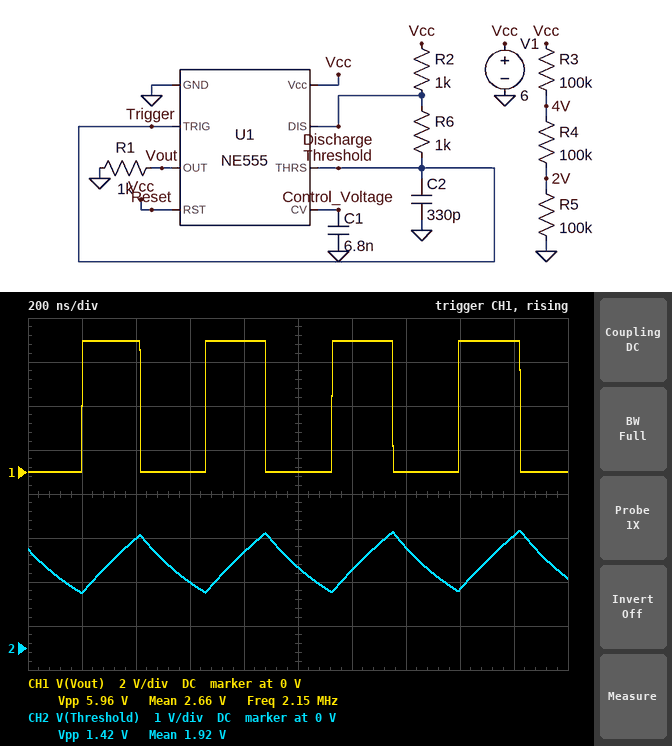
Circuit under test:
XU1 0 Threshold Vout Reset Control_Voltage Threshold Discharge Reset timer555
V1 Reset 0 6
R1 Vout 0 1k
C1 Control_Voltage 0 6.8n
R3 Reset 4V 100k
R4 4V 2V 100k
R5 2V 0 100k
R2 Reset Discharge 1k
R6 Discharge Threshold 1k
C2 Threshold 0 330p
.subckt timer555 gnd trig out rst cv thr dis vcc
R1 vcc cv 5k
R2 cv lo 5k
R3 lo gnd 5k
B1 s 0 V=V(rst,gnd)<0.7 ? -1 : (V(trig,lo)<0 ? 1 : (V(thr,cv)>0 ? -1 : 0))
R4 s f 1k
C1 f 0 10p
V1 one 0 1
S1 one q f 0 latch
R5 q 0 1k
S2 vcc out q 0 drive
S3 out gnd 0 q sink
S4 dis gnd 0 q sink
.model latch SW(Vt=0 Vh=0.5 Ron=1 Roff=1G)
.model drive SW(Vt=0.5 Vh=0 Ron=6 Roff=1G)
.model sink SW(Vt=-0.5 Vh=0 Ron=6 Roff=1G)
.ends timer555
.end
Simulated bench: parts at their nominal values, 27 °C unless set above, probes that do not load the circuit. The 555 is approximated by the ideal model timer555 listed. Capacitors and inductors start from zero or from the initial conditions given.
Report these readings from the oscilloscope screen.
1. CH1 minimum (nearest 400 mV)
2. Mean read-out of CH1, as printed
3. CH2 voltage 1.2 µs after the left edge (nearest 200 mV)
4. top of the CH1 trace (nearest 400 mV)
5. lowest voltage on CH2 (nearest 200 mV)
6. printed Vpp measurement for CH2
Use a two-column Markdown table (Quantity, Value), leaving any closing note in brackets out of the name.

| Quantity | Value |
|---|---|
| CH1 minimum | 0 V |
| Mean read-out of CH1, as printed | 2.66 V |
| CH2 voltage 1.2 µs after the left edge | 1.8 V |
| top of the CH1 trace | 6.0 V |
| lowest voltage on CH2 | 1.2 V |
| printed Vpp measurement for CH2 | 1.42 V |
